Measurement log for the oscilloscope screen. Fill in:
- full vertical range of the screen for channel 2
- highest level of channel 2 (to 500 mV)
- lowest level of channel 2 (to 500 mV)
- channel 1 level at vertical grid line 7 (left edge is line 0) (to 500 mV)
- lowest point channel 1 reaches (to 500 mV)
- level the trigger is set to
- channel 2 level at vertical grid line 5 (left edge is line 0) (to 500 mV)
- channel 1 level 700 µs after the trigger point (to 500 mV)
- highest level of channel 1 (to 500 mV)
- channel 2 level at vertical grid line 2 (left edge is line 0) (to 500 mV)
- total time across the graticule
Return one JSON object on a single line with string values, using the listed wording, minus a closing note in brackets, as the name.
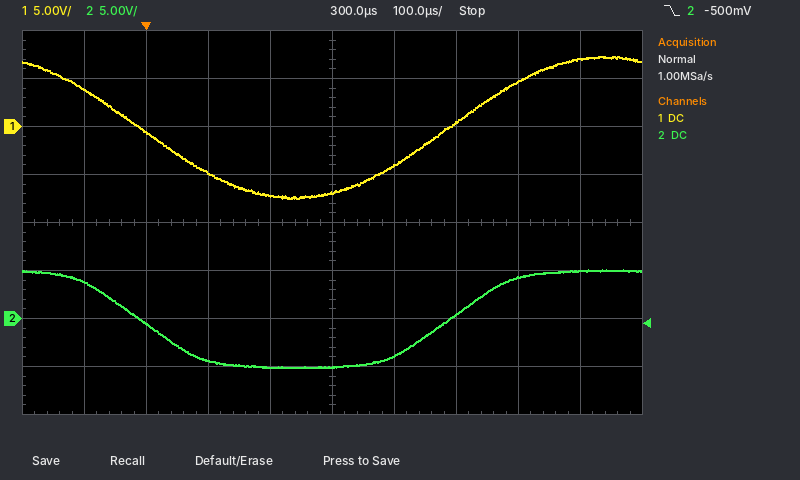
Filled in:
{"full vertical range of the screen for channel 2": "40 V", "highest level of channel 2": "5.0 V", "lowest level of channel 2": "-5.0 V", "channel 1 level at vertical grid line 7 (left edge is line 0)": "500 mV", "lowest point channel 1 reaches": "-7.5 V", "level the trigger is set to": "-500 mV", "channel 2 level at vertical grid line 5 (left edge is line 0)": "-5.0 V", "channel 1 level 700 µs after the trigger point": "7.0 V", "highest level of channel 1": "7.5 V", "channel 2 level at vertical grid line 2 (left edge is line 0)": "-500 mV", "total time across the graticule": "1 ms"}
